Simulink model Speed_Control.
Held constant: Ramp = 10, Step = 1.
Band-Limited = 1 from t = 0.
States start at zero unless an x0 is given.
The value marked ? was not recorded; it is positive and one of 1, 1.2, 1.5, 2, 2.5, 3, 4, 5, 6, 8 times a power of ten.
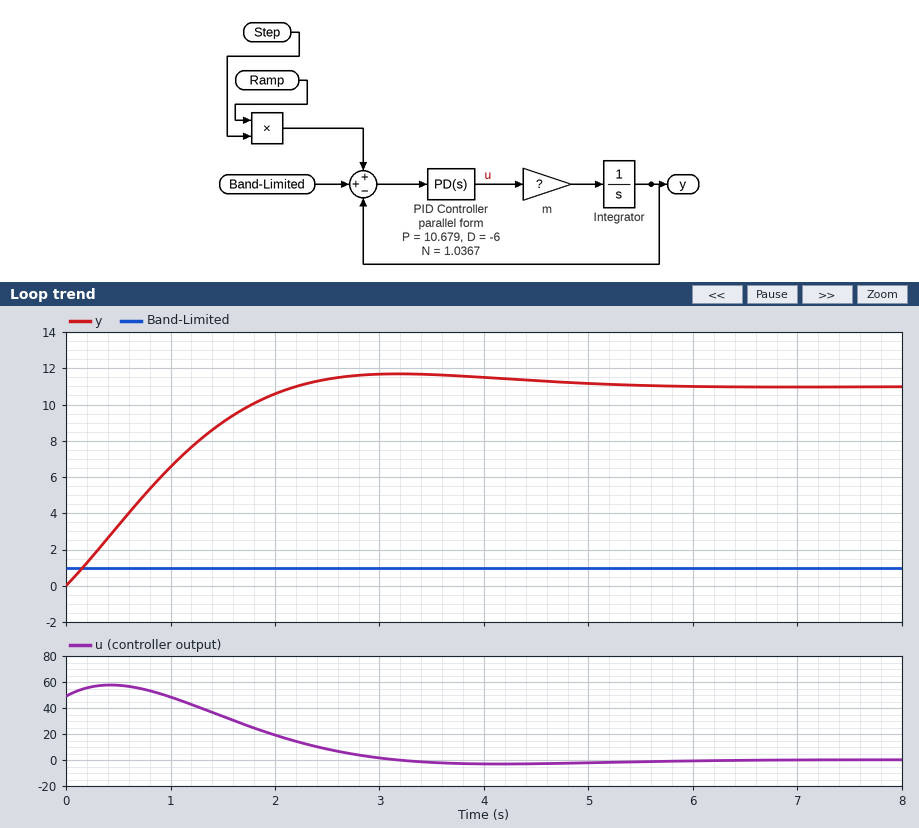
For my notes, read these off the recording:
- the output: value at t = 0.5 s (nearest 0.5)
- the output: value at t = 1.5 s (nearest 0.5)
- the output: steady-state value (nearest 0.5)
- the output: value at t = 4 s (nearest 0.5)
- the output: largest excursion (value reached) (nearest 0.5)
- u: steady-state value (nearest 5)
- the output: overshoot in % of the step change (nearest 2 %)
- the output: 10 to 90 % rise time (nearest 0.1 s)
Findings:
3.5
9.0
11.0
11.5
11.5
0
6 %
1.6 s
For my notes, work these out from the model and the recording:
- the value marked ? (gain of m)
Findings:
0.12
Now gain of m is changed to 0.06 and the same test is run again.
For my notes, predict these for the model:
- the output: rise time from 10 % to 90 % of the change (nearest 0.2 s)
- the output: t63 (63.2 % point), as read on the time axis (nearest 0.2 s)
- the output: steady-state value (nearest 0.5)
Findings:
2.8 s
1.8 s
11.0
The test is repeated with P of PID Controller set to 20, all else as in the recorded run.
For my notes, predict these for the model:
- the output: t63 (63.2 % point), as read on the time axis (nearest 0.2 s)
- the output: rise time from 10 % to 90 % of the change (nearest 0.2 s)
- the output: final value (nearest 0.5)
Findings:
0.6 s
1.0 s
11.0
